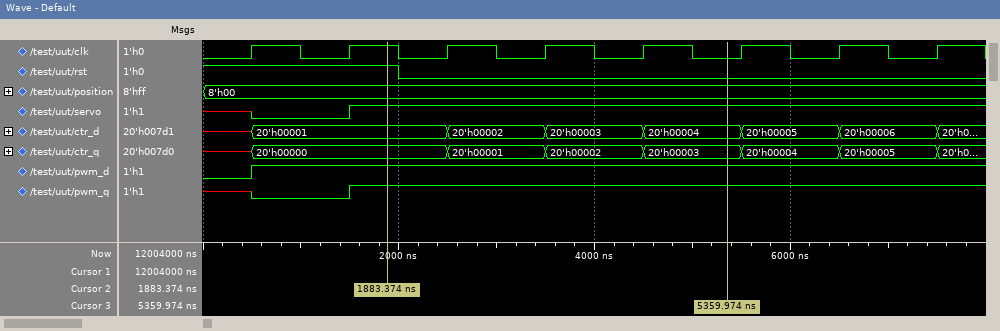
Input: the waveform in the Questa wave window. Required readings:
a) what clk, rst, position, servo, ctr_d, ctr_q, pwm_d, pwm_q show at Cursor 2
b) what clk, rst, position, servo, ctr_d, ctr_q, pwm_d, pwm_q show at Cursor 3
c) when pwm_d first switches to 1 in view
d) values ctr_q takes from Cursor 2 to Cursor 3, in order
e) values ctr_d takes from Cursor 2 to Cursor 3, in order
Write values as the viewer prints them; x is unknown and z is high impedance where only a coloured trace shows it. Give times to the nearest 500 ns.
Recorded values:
clk=1, rst=1, position=8'h00, servo=1, ctr_d=20'h00001, ctr_q=20'h00000, pwm_d=1, pwm_q=1
clk=0, rst=0, position=8'h00, servo=1, ctr_d=20'h00004, ctr_q=20'h00003, pwm_d=1, pwm_q=1
500 ns
20'h00000, 20'h00001, 20'h00002, 20'h00003
20'h00001, 20'h00002, 20'h00003, 20'h00004
